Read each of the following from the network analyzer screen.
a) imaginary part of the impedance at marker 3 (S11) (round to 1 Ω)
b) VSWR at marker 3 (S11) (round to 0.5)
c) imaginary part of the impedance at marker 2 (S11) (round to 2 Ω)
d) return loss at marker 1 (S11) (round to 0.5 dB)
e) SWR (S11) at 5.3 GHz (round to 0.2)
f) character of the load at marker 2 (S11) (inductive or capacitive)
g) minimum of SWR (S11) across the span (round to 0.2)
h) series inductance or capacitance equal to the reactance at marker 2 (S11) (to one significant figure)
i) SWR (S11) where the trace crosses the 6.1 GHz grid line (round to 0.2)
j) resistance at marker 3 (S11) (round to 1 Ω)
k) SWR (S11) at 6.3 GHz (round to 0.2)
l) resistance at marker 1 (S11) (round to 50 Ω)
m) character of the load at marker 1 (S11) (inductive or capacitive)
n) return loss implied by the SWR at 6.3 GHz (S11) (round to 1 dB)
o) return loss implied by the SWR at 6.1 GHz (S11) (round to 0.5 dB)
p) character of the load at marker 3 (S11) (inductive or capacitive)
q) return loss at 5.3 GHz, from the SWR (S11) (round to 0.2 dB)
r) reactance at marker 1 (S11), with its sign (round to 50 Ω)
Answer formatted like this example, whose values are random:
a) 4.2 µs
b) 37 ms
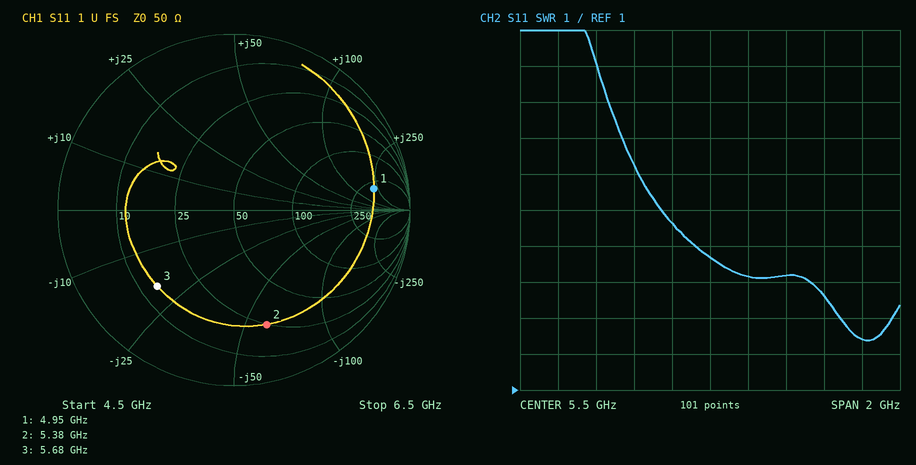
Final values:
a) -19 Ω
b) 4.0
c) -60 Ω
d) 2.0 dB
e) 5.6
f) capacitive
g) 2.4
h) 500 fF
i) 3.6
j) 14 Ω
k) 2.4
l) 300 Ω
m) inductive
n) 8 dB
o) 5.0 dB
p) capacitive
q) 3.2 dB
r) +200 Ω
